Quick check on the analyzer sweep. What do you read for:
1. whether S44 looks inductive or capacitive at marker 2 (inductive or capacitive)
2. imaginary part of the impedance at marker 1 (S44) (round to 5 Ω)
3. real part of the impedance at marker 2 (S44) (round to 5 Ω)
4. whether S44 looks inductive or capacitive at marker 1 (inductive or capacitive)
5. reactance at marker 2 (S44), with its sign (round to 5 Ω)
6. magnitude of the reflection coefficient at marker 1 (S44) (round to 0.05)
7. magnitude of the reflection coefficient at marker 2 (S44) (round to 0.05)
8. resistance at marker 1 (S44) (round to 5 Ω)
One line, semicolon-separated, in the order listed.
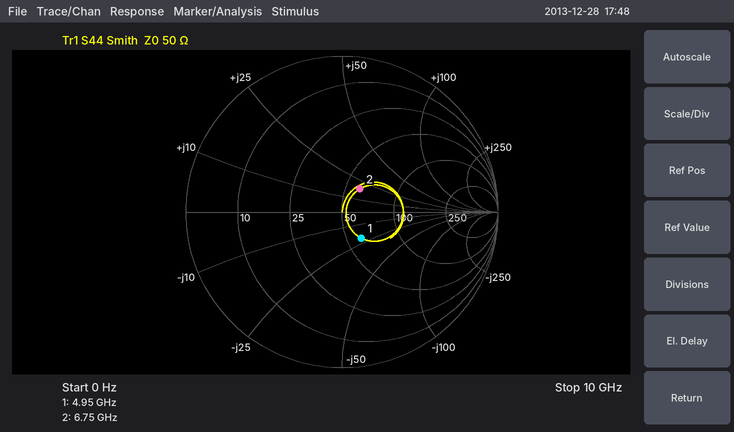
inductive; -20 Ω; 60 Ω; capacitive; +20 Ω; 0.20; 0.20; 60 Ω
